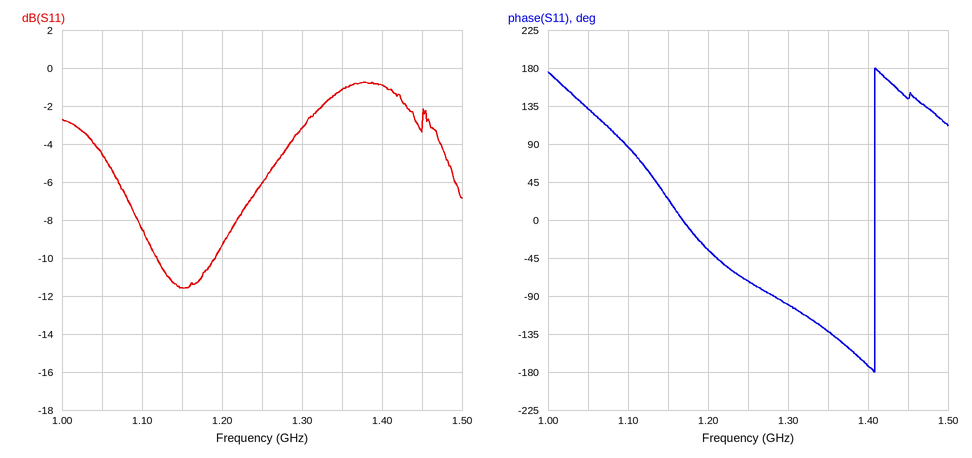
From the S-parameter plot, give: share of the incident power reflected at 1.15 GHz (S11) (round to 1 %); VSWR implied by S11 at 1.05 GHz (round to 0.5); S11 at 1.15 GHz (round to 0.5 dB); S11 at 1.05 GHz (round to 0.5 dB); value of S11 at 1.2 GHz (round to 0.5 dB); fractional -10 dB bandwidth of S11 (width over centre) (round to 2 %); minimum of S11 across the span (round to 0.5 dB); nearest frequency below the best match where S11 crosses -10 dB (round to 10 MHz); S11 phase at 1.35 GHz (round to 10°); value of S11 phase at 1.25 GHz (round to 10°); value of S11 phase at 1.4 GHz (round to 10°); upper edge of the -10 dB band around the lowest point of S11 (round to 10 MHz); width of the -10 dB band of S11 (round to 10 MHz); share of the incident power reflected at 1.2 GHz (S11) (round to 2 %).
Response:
7 %
4.0
-11.5 dB
-4.5 dB
-9.5 dB
6 %
-11.5 dB
1.12 GHz
-130°
-70°
-170°
1.19 GHz
70 MHz
12 %
